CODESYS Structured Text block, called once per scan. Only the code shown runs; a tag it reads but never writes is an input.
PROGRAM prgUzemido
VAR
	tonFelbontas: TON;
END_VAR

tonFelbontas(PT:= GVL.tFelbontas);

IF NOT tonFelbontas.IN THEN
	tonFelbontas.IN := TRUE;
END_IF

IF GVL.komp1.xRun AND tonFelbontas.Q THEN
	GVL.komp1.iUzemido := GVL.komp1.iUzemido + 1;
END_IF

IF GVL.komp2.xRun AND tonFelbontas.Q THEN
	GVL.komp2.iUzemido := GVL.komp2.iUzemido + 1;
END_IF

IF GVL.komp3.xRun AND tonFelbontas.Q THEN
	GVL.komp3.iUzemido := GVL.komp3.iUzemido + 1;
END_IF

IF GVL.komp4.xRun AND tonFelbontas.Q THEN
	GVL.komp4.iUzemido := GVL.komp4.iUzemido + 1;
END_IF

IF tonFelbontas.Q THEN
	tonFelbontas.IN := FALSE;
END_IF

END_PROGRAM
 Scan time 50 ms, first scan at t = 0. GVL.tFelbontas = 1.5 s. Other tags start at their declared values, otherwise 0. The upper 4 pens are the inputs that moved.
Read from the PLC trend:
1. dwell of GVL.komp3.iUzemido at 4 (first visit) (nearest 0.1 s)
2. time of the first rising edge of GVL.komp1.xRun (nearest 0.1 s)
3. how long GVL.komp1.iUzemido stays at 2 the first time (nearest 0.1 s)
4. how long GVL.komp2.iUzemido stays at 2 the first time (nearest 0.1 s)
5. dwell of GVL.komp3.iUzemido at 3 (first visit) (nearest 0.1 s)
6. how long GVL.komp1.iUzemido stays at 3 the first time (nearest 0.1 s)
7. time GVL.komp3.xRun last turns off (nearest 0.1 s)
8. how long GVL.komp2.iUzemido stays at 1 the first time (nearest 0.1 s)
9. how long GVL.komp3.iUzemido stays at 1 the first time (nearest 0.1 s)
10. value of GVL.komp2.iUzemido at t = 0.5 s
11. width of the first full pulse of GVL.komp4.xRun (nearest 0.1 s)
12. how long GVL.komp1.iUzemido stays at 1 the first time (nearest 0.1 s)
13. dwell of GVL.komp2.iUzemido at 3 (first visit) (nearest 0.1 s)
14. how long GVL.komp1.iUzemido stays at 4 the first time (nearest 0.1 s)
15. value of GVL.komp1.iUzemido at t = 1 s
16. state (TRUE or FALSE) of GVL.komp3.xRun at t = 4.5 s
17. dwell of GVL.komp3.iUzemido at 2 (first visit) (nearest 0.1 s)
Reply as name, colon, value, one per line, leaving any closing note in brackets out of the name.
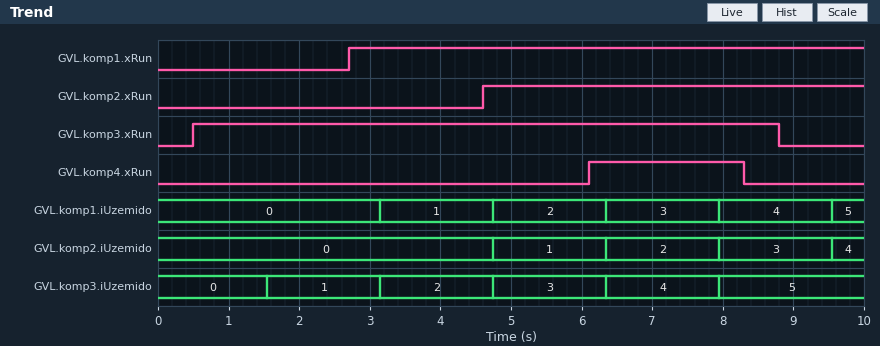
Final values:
dwell of GVL.komp3.iUzemido at 4 (first visit): 1.6 s
time of the first rising edge of GVL.komp1.xRun: 2.7 s
how long GVL.komp1.iUzemido stays at 2 the first time: 1.6 s
how long GVL.komp2.iUzemido stays at 2 the first time: 1.6 s
dwell of GVL.komp3.iUzemido at 3 (first visit): 1.6 s
how long GVL.komp1.iUzemido stays at 3 the first time: 1.6 s
time GVL.komp3.xRun last turns off: 8.8 s
how long GVL.komp2.iUzemido stays at 1 the first time: 1.6 s
how long GVL.komp3.iUzemido stays at 1 the first time: 1.6 s
value of GVL.komp2.iUzemido at t = 0.5 s: 0
width of the first full pulse of GVL.komp4.xRun: 2.2 s
how long GVL.komp1.iUzemido stays at 1 the first time: 1.6 s
dwell of GVL.komp2.iUzemido at 3 (first visit): 1.6 s
how long GVL.komp1.iUzemido stays at 4 the first time: 1.6 s
value of GVL.komp1.iUzemido at t = 1 s: 0
state (TRUE or FALSE) of GVL.komp3.xRun at t = 4.5 s: TRUE
dwell of GVL.komp3.iUzemido at 2 (first visit): 1.6 s
